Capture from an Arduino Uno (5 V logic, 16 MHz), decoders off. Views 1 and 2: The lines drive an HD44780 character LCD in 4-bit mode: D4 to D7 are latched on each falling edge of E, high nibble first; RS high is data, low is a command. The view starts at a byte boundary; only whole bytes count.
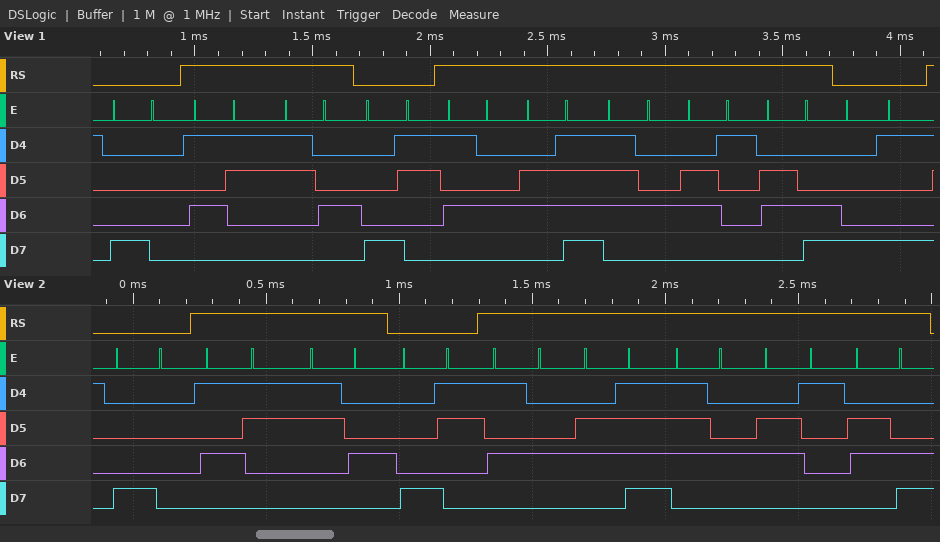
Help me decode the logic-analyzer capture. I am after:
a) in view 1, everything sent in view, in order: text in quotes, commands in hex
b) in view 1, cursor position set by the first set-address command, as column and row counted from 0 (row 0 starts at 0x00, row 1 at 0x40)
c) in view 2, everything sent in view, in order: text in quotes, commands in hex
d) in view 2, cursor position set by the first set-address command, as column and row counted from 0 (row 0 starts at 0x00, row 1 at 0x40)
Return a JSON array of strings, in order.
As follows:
["0x80 \"S4\" 0x83 \"Total\" 0x89", "column 0, row 0", "0x80 \"S4\" 0x83 \"Total\"", "column 0, row 0"]
